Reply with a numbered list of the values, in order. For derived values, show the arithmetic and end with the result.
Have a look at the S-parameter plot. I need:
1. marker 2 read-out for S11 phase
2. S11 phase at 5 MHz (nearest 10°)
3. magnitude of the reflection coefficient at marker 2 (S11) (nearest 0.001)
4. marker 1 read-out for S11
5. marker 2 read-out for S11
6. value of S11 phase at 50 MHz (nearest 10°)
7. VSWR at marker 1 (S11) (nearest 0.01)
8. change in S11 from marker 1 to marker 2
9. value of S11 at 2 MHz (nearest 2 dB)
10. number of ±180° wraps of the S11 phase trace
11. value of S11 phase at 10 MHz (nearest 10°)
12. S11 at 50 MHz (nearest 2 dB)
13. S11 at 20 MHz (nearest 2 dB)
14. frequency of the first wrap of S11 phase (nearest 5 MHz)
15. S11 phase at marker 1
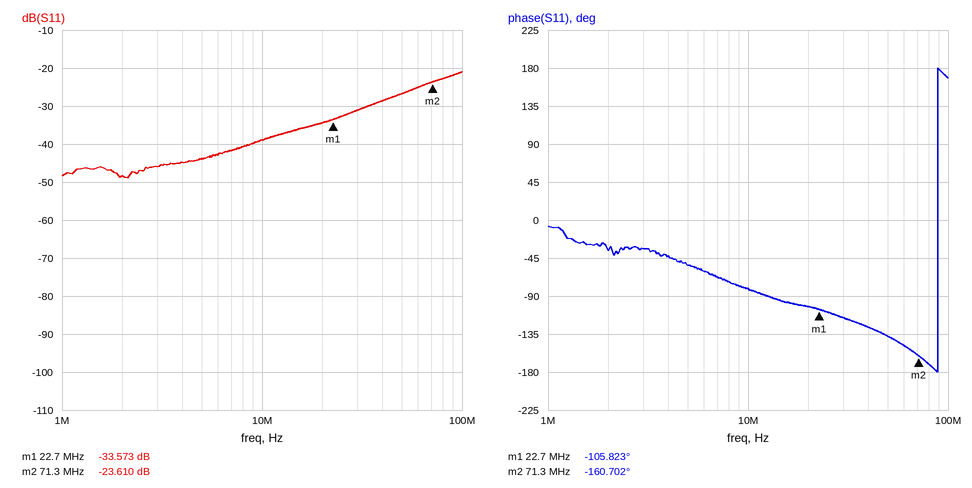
1. -160.702°
2. -50°
3. 10^(-23.61/20) ≈ 0.066
4. -33.573 dB
5. -23.610 dB
6. -140°
7. (1 + 0.0210)/(1 − 0.0210) ≈ 1.04
8. -23.61 − (-33.573) = 9.963 dB
9. -48 dB
10. 1
11. -80°
12. -26 dB
13. -34 dB
14. 90 MHz
15. -105.823°
